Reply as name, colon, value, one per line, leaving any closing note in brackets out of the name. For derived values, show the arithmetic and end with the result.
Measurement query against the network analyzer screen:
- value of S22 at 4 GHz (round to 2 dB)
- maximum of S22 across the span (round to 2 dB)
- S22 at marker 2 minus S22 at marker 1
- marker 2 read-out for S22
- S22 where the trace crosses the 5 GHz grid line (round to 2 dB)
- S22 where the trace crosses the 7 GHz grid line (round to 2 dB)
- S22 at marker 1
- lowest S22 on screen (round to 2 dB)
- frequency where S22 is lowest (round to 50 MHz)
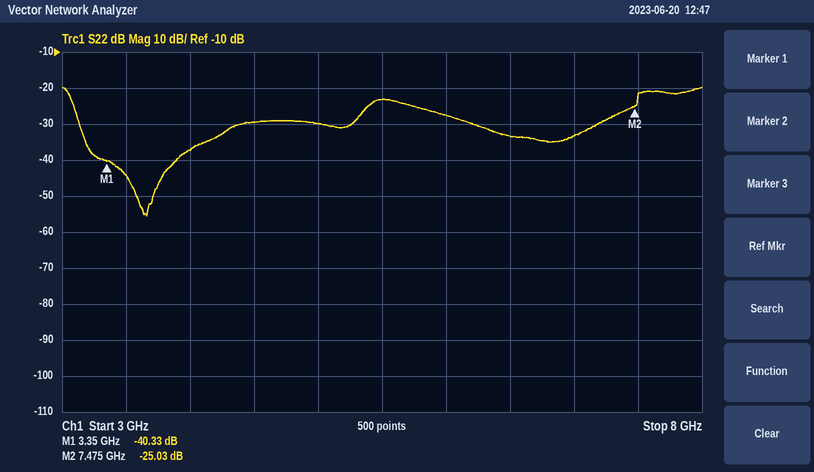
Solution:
value of S22 at 4 GHz: -38 dB
maximum of S22 across the span: -20 dB
S22 at marker 2 minus S22 at marker 1: -25.03 − (-40.33) = 15.30 dB
marker 2 read-out for S22: -25.03 dB
S22 where the trace crosses the 5 GHz grid line: -30 dB
S22 where the trace crosses the 7 GHz grid line: -34 dB
S22 at marker 1: -40.33 dB
lowest S22 on screen: -56 dB
frequency where S22 is lowest: 3.65 GHz
